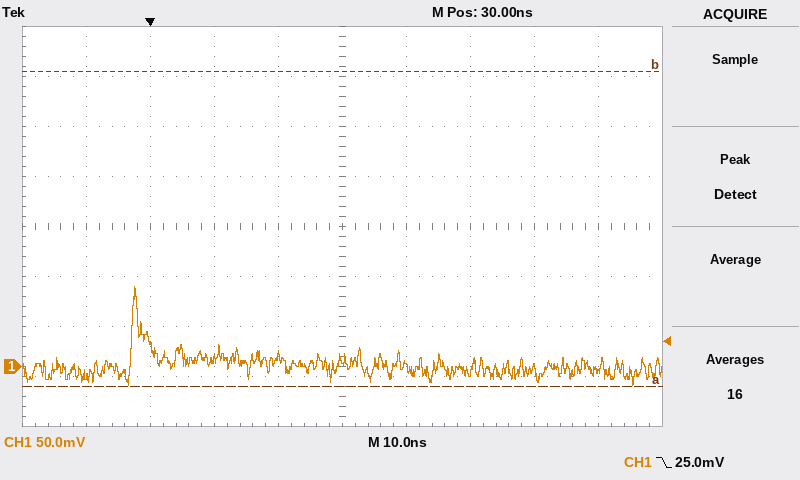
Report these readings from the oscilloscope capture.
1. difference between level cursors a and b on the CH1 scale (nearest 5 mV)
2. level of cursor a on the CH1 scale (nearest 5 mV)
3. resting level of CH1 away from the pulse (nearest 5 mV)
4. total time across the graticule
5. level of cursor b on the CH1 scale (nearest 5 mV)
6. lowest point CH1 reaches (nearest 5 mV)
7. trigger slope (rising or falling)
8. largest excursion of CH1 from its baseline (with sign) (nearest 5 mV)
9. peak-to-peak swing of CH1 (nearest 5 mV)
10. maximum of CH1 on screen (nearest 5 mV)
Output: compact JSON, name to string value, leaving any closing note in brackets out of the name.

{"difference between level cursors a and b on the CH1 scale": "315 mV", "level of cursor a on the CH1 scale": "-20 mV", "resting level of CH1 away from the pulse": "0 mV", "total time across the graticule": "100 ns", "level of cursor b on the CH1 scale": "295 mV", "lowest point CH1 reaches": "-20 mV", "trigger slope": "falling", "largest excursion of CH1 from its baseline (with sign)": "+80 mV", "peak-to-peak swing of CH1": "100 mV", "maximum of CH1 on screen": "80 mV"}
